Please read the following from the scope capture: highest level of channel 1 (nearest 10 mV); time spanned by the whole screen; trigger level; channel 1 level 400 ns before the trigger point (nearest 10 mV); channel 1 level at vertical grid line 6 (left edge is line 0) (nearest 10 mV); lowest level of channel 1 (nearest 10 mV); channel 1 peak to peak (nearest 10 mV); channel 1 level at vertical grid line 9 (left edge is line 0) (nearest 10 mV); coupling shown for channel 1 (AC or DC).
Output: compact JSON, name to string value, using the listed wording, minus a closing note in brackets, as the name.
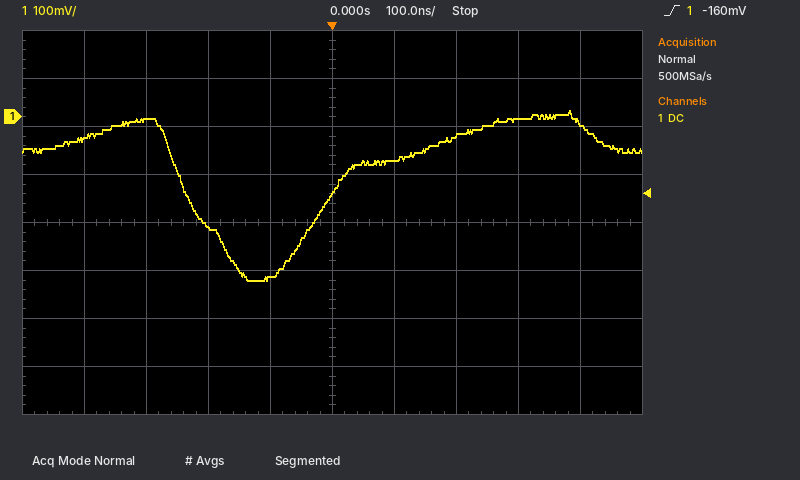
{"highest level of channel 1": "10 mV", "time spanned by the whole screen": "1 µs", "trigger level": "-160 mV", "channel 1 level 400 ns before the trigger point": "-50 mV", "channel 1 level at vertical grid line 6 (left edge is line 0)": "-90 mV", "lowest level of channel 1": "-340 mV", "channel 1 peak to peak": "350 mV", "channel 1 level at vertical grid line 9 (left edge is line 0)": "-10 mV", "coupling shown for channel 1": "DC"}
